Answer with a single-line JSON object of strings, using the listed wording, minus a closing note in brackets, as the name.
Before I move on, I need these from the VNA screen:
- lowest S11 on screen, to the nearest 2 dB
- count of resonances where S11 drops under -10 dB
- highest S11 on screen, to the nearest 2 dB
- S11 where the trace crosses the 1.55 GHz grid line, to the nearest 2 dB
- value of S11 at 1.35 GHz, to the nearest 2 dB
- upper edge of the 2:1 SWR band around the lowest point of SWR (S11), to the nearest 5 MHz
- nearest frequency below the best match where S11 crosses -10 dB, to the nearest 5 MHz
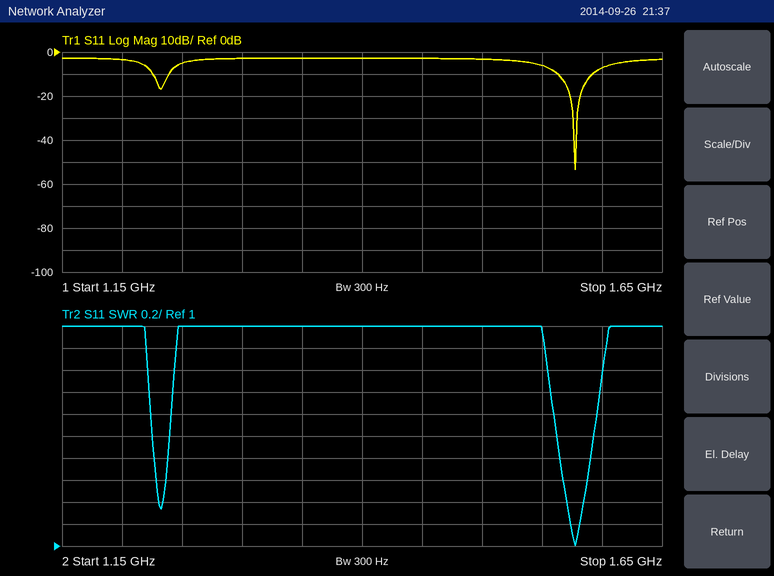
{"lowest S11 on screen, to the nearest 2 dB": "-54 dB", "count of resonances where S11 drops under -10 dB": "2", "highest S11 on screen, to the nearest 2 dB": "-2 dB", "S11 where the trace crosses the 1.55 GHz grid line, to the nearest 2 dB": "-6 dB", "value of S11 at 1.35 GHz, to the nearest 2 dB": "-2 dB", "upper edge of the 2:1 SWR band around the lowest point of SWR (S11), to the nearest 5 MHz": "1.595 GHz", "nearest frequency below the best match where S11 crosses -10 dB, to the nearest 5 MHz": "1.565 GHz"}
